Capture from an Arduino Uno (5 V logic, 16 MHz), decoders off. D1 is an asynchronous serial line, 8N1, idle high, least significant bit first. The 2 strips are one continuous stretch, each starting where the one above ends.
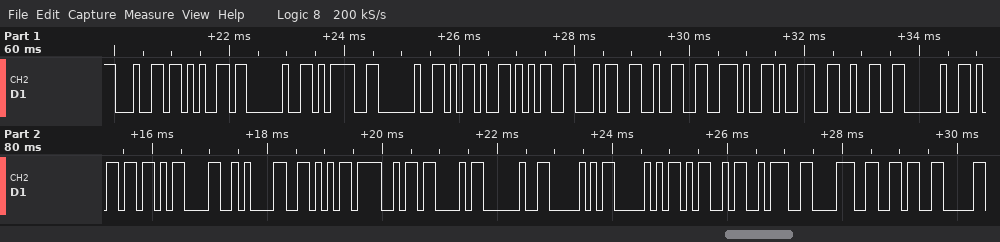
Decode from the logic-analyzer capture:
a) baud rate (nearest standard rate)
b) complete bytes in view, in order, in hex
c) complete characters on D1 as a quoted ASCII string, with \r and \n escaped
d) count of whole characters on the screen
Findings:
9600 baud
64 65 20 3D 20 2D 35 34 32 2E 39 32 20 6D 0D 0A 56 4F 43 20 50 50 4D 3A 38 36
"de = -542.92 m\r\nVOC PPM:86"
26
